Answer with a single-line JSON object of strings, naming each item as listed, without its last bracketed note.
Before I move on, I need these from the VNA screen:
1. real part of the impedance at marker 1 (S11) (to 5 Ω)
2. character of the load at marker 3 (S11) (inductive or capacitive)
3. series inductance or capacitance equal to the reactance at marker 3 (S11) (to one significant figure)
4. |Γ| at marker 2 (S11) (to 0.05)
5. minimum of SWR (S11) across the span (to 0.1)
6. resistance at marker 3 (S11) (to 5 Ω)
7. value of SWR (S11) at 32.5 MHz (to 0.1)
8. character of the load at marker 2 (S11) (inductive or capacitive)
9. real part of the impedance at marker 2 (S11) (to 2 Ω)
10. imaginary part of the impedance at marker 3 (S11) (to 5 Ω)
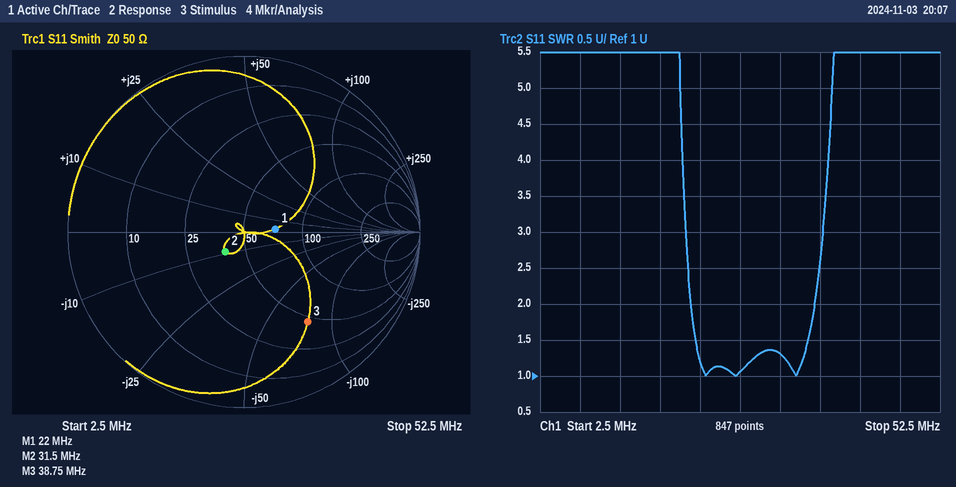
{"real part of the impedance at marker 1 (S11)": "70 Ω", "character of the load at marker 3 (S11)": "capacitive", "series inductance or capacitance equal to the reactance at marker 3 (S11)": "50 pF", "|Γ| at marker 2 (S11)": "0.15", "minimum of SWR (S11) across the span": "1.0", "resistance at marker 3 (S11)": "45 Ω", "value of SWR (S11) at 32.5 MHz": "1.3", "character of the load at marker 2 (S11)": "capacitive", "real part of the impedance at marker 2 (S11)": "40 Ω", "imaginary part of the impedance at marker 3 (S11)": "-75 Ω"}
